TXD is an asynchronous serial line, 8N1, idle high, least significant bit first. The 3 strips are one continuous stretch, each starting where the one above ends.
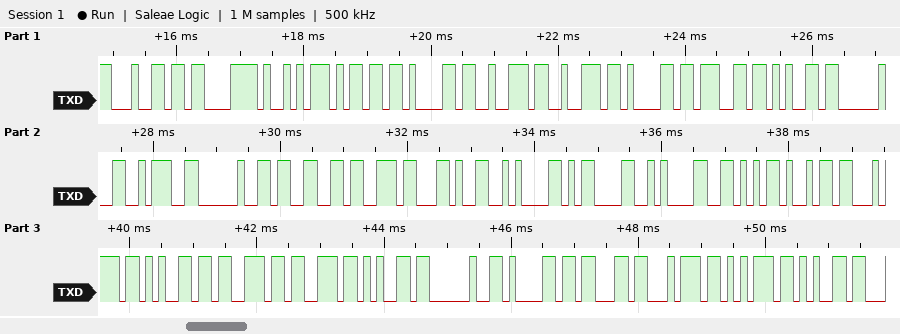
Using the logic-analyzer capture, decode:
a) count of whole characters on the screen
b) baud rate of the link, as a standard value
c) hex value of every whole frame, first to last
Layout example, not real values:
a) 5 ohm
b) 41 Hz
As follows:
a) 32
b) 9600 baud
c) 64 C3 A9 6D 61 72 72 61 67 65 20 3A 20 33 73 2C 0A 0D 0A 56 69 74 65 73 73 65 20 61 63 74 75 65
